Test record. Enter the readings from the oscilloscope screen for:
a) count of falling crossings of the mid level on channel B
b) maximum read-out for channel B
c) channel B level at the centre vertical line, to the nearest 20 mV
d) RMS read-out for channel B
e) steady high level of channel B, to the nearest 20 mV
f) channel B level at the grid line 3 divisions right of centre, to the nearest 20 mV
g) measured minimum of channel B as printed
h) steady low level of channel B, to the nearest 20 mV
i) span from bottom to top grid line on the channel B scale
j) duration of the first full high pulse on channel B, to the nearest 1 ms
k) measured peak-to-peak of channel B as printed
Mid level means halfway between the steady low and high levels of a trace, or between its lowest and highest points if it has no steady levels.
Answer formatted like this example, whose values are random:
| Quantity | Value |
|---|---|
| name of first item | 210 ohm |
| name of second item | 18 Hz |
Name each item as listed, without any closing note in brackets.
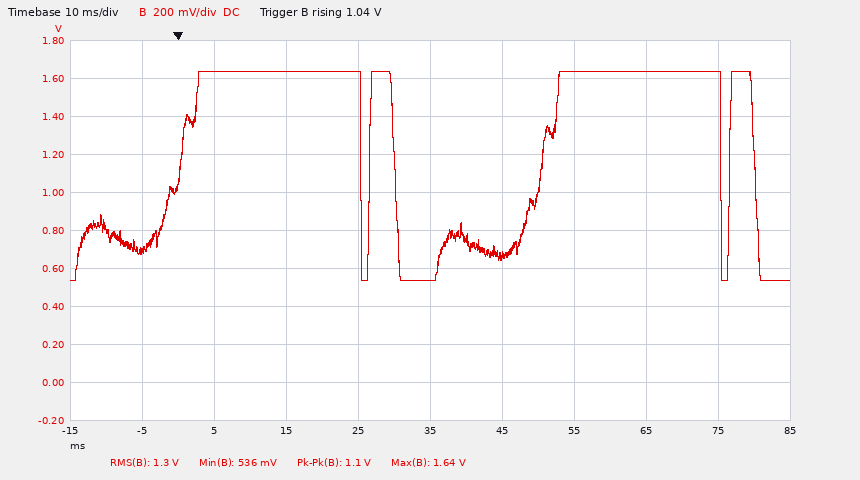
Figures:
| Quantity | Value |
|---|---|
| count of falling crossings of the mid level on channel B | 4 |
| maximum read-out for channel B | 1.64 V |
| channel B level at the centre vertical line, to the nearest 20 mV | 540 mV |
| RMS read-out for channel B | 1.3 V |
| steady high level of channel B, to the nearest 20 mV | 1.64 V |
| channel B level at the grid line 3 divisions right of centre, to the nearest 20 mV | 1.64 V |
| measured minimum of channel B as printed | 536 mV |
| steady low level of channel B, to the nearest 20 mV | 540 mV |
| span from bottom to top grid line on the channel B scale | 2 V |
| duration of the first full high pulse on channel B, to the nearest 1 ms | 25 ms |
| measured peak-to-peak of channel B as printed | 1.1 V |
